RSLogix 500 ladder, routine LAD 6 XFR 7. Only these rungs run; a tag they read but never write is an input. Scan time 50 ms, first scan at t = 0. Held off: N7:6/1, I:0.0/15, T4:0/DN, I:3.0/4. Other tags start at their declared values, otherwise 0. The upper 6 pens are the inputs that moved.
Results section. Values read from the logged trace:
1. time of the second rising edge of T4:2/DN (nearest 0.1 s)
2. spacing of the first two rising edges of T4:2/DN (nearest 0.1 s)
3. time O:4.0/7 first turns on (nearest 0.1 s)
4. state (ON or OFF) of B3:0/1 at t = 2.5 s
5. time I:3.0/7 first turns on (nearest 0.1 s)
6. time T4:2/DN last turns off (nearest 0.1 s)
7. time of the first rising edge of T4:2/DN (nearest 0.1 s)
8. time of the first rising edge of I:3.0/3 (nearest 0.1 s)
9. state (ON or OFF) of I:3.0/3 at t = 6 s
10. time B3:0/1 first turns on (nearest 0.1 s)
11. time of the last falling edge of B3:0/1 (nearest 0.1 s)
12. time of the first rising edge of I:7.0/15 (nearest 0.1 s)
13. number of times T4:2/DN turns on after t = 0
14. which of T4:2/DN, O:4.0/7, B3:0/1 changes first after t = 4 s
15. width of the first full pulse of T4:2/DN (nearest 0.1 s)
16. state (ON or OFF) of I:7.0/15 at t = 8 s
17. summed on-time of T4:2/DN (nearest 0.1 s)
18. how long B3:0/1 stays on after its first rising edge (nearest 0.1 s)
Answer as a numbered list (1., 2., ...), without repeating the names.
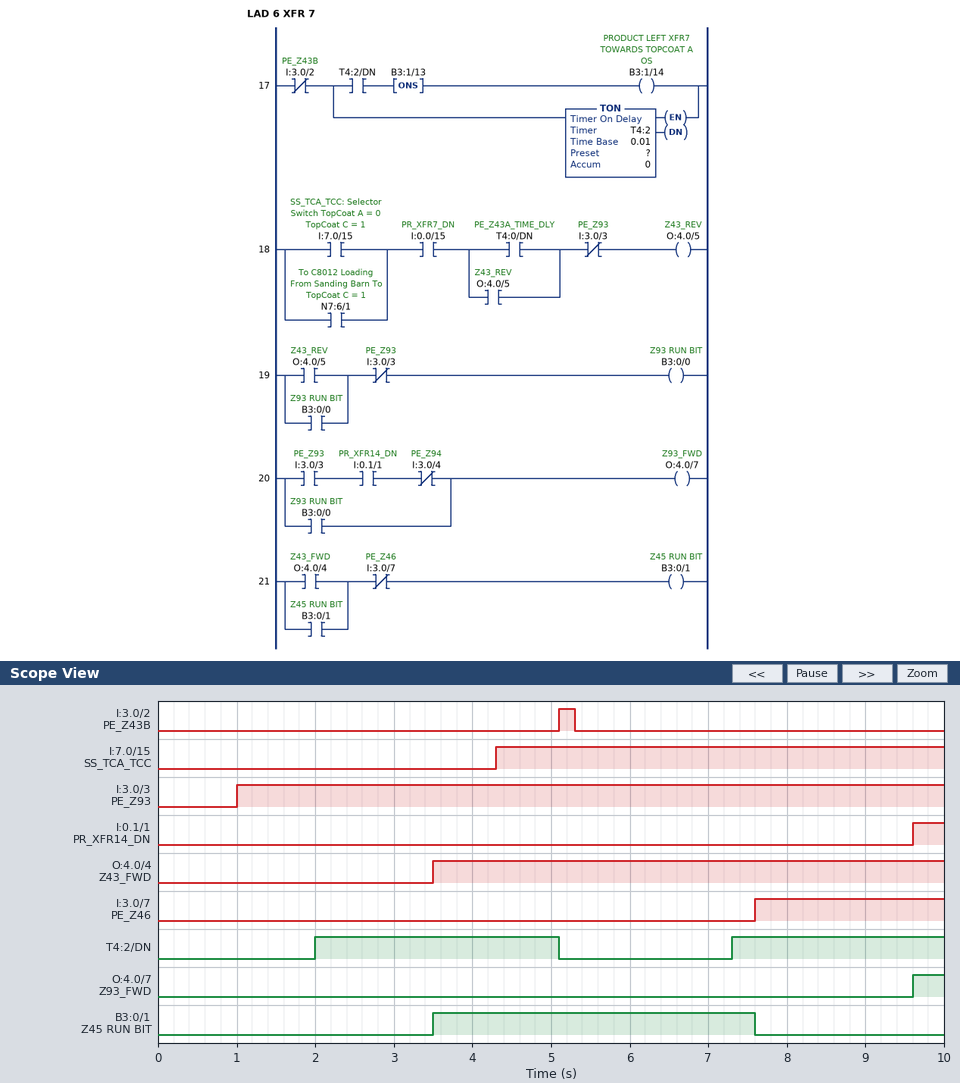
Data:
1. 7.3 s
2. 5.3 s
3. 9.6 s
4. OFF
5. 7.6 s
6. 5.1 s
7. 2.0 s
8. 1.0 s
9. ON
10. 3.5 s
11. 7.6 s
12. 4.3 s
13. 2
14. T4:2/DN
15. 3.1 s
16. ON
17. 5.8 s
18. 4.1 s
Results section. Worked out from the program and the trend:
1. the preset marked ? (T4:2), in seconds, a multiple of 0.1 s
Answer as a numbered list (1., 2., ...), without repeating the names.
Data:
1. 2.0 s
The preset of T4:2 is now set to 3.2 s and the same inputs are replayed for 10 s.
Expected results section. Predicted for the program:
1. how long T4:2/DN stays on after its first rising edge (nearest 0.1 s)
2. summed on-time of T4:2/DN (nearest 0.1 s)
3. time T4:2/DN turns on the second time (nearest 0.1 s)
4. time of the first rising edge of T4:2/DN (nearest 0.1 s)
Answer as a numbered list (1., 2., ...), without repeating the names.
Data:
1. 1.9 s
2. 3.4 s
3. 8.5 s
4. 3.2 s
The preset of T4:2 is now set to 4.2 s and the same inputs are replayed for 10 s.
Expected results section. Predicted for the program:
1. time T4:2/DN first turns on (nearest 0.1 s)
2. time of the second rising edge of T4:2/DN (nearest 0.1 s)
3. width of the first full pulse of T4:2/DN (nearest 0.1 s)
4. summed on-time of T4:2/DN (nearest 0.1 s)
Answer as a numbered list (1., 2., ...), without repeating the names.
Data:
1. 4.2 s
2. 9.5 s
3. 0.9 s
4. 1.4 s
